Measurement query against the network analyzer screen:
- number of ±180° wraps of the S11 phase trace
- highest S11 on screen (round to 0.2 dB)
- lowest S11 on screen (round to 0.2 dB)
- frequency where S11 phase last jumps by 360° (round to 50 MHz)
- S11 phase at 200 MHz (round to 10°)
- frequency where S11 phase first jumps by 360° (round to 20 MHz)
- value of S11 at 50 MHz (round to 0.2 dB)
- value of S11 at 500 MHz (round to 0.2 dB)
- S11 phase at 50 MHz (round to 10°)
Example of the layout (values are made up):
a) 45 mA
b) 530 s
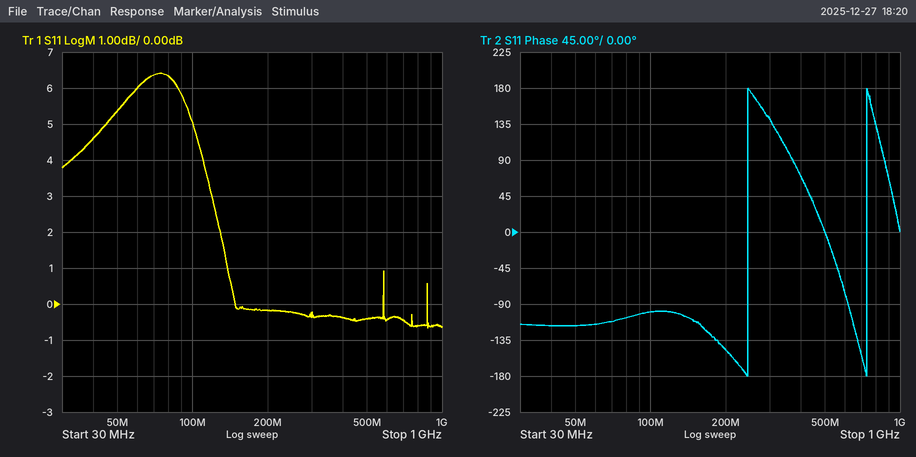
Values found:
a) 2
b) 6.4 dB
c) -0.6 dB
d) 750 MHz
e) -150°
f) 240 MHz
g) 5.4 dB
h) -0.4 dB
i) -120°
